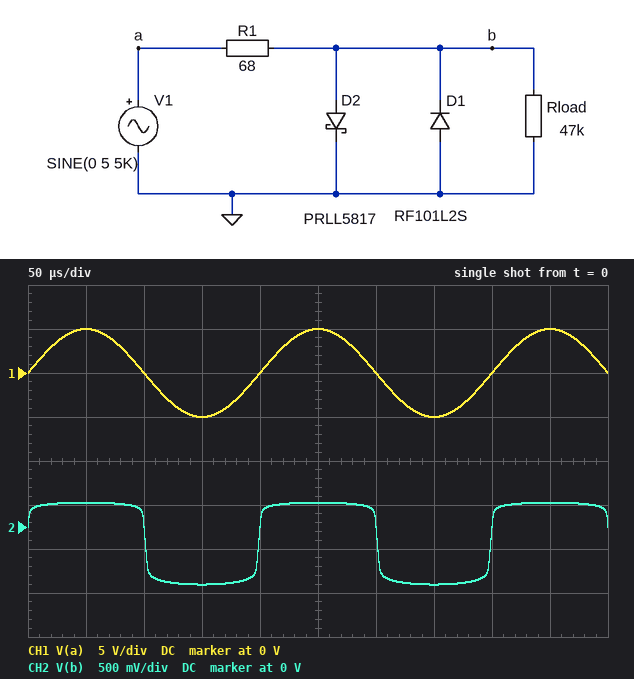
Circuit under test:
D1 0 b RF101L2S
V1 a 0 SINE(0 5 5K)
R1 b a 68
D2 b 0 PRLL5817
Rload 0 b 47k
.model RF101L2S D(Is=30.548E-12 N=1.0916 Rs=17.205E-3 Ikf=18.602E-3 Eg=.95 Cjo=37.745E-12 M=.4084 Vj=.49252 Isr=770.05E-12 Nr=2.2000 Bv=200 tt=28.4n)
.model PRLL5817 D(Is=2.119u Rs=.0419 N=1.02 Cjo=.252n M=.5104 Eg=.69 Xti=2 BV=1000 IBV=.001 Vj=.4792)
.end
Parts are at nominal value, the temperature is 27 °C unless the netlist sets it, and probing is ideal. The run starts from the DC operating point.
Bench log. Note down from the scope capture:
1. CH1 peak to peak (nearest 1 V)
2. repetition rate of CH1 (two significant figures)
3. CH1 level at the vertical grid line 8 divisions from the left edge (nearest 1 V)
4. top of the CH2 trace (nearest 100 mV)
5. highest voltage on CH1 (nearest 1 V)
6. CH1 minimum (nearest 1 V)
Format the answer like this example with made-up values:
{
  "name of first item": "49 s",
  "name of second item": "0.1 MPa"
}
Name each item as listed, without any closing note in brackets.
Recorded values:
{
  "CH1 peak to peak": "10 V",
  "repetition rate of CH1": "5.0 kHz",
  "CH1 level at the vertical grid line 8 divisions from the left edge": "0 V",
  "top of the CH2 trace": "300 mV",
  "highest voltage on CH1": "5 V",
  "CH1 minimum": "-5 V"
}
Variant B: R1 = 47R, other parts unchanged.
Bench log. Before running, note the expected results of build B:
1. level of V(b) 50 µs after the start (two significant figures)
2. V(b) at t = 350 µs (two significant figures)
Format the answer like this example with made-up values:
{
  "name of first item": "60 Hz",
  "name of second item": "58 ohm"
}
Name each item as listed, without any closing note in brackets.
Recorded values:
{
  "level of V(b) 50 µs after the start": "290 mV",
  "V(b) at t = 350 µs": "-670 mV"
}
